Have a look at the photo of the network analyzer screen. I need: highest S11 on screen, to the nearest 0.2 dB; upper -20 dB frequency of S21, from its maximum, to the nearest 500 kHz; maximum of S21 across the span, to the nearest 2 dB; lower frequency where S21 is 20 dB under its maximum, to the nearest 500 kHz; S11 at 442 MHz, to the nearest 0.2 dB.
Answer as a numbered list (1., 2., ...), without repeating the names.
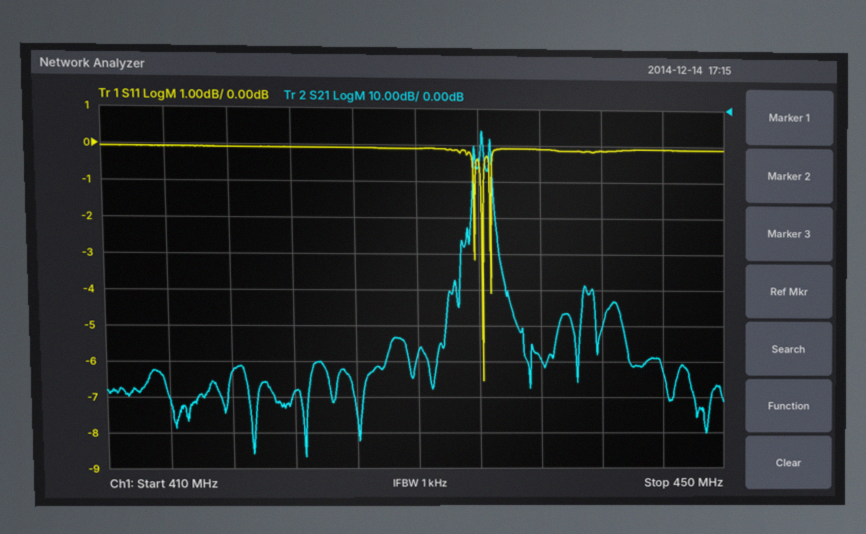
1. 0.0 dB
2. 435.0 MHz
3. -6 dB
4. 433.5 MHz
5. -0.2 dB
